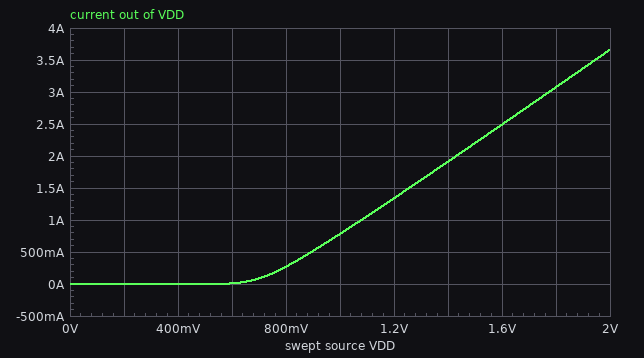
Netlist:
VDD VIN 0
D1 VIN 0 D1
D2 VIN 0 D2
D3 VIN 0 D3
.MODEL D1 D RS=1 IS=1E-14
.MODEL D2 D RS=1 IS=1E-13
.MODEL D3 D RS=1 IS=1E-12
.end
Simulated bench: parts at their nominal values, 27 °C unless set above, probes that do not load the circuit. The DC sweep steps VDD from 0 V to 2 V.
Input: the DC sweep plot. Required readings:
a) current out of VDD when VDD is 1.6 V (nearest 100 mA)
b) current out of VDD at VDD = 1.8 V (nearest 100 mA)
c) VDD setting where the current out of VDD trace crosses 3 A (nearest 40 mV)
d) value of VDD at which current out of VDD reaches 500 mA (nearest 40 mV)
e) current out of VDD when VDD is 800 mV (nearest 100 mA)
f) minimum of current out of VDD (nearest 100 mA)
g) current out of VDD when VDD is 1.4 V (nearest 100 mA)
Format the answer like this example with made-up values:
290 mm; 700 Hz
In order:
2.5 A; 3.1 A; 1.76 V; 880 mV; 300 mA; 0 A; 1.9 A
